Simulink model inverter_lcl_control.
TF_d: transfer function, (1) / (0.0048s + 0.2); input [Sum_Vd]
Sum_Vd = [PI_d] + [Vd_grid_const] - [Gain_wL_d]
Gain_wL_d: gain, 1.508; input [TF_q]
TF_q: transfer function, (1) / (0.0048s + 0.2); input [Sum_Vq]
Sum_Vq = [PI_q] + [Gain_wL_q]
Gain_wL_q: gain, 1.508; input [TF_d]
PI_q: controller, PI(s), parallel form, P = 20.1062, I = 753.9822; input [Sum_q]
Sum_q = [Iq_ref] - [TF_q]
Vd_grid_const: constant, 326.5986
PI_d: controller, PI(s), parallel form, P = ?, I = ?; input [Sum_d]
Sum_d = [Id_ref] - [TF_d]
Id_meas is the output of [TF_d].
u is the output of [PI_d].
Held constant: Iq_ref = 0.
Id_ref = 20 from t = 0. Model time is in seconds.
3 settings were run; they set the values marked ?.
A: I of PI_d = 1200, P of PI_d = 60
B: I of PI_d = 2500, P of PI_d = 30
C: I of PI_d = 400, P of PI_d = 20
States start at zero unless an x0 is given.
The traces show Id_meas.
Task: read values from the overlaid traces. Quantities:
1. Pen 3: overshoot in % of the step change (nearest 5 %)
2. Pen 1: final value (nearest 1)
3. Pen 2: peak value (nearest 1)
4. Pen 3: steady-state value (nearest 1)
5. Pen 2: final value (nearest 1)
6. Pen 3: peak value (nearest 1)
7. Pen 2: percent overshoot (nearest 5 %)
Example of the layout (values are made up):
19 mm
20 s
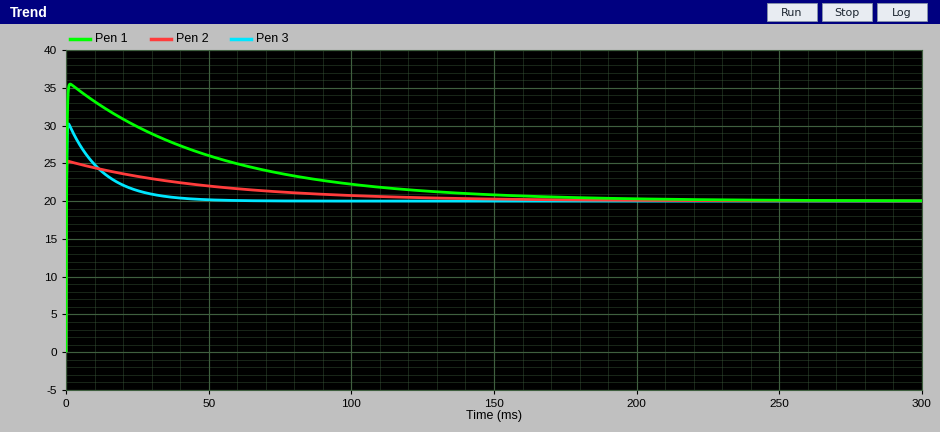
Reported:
50 %
20
25
20
20
30
25 %
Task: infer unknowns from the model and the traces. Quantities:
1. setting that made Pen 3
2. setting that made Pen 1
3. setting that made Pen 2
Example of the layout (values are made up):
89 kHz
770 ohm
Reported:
B
C
A
